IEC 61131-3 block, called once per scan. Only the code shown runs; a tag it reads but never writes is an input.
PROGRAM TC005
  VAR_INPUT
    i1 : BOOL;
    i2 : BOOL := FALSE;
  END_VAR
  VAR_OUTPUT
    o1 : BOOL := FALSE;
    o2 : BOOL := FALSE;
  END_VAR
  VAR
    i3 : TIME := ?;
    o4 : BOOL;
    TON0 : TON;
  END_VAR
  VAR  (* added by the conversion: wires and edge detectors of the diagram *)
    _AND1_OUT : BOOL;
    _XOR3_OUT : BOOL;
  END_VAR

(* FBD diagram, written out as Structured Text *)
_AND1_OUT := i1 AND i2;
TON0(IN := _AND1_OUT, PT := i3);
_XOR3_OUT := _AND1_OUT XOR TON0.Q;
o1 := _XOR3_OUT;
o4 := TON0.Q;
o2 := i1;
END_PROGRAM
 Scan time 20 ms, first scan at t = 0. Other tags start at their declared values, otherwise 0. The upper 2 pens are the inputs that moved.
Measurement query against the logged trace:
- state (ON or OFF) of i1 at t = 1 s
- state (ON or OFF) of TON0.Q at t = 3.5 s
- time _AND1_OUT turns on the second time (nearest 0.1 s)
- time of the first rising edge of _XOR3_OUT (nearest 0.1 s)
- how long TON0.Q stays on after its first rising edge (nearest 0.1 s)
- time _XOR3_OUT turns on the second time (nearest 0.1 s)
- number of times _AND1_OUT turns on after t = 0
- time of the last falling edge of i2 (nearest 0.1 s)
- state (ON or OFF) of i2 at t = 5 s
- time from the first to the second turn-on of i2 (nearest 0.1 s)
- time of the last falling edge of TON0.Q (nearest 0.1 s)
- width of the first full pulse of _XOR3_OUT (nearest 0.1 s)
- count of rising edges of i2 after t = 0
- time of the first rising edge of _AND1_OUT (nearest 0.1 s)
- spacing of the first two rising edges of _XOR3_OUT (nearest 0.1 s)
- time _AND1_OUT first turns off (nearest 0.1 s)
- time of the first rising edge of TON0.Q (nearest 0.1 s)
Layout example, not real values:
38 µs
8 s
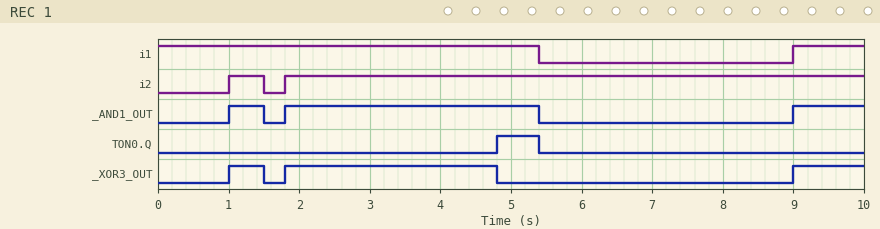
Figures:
ON
OFF
1.8 s
1.0 s
0.6 s
1.8 s
3
1.5 s
ON
0.8 s
5.4 s
0.5 s
2
1.0 s
0.8 s
1.5 s
4.8 s
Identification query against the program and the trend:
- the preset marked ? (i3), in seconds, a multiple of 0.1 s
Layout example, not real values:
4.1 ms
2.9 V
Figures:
3.0 s
